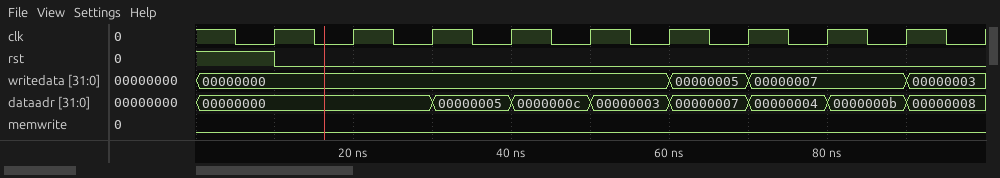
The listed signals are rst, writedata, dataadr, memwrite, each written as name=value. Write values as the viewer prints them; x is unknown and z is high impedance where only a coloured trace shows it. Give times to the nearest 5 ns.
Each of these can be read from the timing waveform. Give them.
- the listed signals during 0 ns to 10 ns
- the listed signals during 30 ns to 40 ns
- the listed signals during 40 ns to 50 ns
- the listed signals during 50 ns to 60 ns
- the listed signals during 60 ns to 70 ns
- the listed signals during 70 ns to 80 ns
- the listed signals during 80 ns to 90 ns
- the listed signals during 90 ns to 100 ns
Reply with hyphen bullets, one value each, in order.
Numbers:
- rst=1, writedata=00000000, dataadr=00000000, memwrite=0
- rst=0, writedata=00000000, dataadr=00000005, memwrite=0
- rst=0, writedata=00000000, dataadr=0000000c, memwrite=0
- rst=0, writedata=00000000, dataadr=00000003, memwrite=0
- rst=0, writedata=00000005, dataadr=00000007, memwrite=0
- rst=0, writedata=00000007, dataadr=00000004, memwrite=0
- rst=0, writedata=00000007, dataadr=0000000b, memwrite=0
- rst=0, writedata=00000003, dataadr=00000008, memwrite=0
